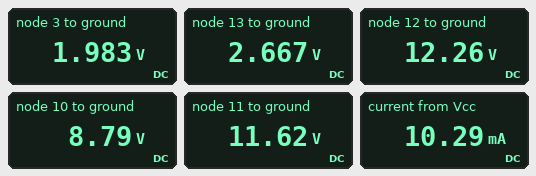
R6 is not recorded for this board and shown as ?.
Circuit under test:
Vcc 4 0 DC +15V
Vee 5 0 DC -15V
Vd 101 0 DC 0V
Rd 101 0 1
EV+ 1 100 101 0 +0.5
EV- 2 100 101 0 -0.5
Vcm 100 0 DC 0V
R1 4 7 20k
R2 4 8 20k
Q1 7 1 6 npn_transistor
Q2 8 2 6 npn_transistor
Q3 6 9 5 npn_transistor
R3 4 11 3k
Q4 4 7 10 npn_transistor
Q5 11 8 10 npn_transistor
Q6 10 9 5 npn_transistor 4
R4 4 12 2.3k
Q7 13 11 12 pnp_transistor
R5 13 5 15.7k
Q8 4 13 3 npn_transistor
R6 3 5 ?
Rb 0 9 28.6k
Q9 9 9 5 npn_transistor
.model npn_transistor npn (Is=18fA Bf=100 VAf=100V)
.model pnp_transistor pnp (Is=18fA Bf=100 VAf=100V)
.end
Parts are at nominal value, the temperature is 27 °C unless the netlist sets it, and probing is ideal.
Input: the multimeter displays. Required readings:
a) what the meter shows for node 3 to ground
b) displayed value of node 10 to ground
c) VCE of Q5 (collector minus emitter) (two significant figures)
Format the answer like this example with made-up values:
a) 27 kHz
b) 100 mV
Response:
a) 1.983 V
b) 8.79 V
c) 2.8 V
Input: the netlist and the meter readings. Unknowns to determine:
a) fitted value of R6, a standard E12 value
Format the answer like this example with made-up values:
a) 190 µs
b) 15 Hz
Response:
a) 2.7 kΩ
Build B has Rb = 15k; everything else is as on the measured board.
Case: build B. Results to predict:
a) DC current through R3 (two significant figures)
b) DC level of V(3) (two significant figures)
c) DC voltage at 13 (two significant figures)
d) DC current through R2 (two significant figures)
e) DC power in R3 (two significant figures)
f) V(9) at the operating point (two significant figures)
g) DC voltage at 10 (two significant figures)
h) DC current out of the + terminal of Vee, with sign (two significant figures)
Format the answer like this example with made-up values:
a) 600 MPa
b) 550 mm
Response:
a) 1.8 mA
b) 9.6 V
c) 10 V
d) 530 µA
e) 9.3 mW
f) -14 V
g) 3.8 V
h) -17 mA
